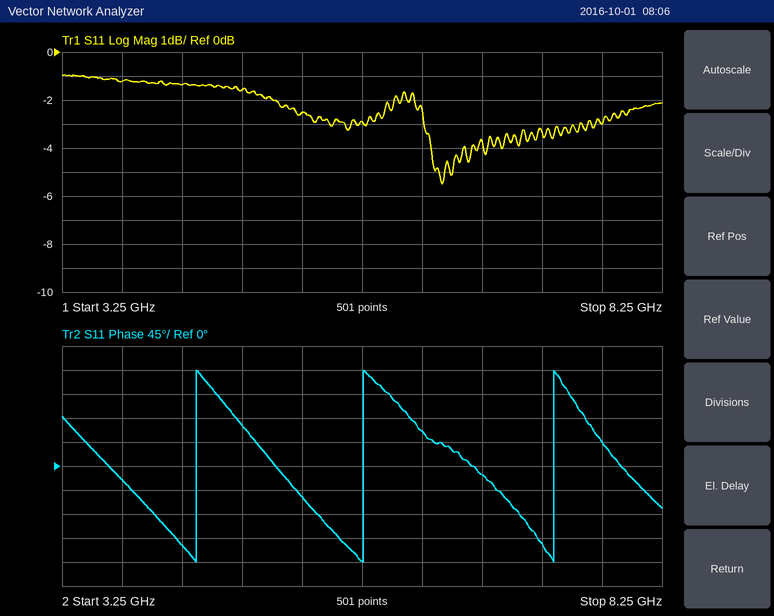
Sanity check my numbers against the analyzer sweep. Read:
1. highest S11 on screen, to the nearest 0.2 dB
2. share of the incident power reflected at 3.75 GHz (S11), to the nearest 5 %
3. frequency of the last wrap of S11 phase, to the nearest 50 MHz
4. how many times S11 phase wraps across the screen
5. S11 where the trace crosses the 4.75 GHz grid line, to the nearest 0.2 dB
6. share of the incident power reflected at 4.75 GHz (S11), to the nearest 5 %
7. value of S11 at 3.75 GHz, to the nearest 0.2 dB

-1.0 dB
75 %
7.35 GHz
3
-1.6 dB
70 %
-1.2 dB
